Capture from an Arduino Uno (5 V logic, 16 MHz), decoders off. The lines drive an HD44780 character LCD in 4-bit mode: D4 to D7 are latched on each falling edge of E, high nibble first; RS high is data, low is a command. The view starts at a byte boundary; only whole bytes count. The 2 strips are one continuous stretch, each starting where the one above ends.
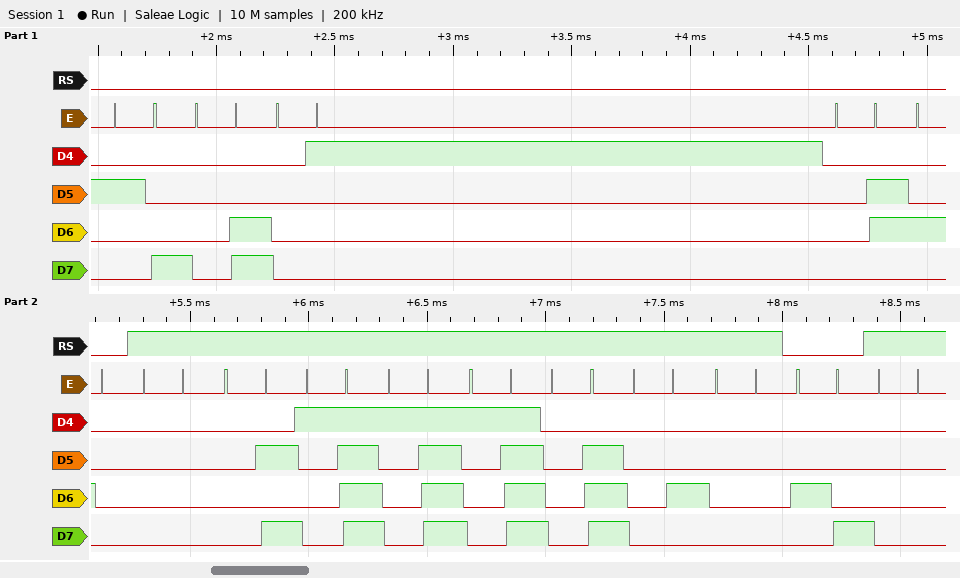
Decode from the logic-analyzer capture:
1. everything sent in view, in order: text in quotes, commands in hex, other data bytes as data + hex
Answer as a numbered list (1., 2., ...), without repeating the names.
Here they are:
1. 0x28 0x0C 0x01 0x06 0x40 data 00 0A 1F 1F 1F 0E 04 00 0x48 data 00
